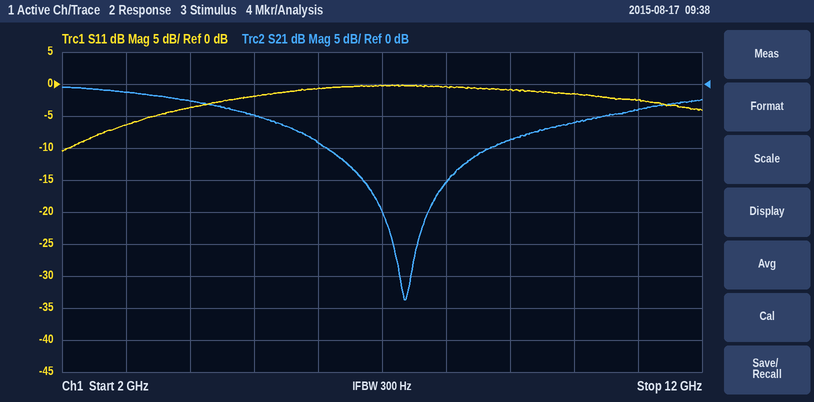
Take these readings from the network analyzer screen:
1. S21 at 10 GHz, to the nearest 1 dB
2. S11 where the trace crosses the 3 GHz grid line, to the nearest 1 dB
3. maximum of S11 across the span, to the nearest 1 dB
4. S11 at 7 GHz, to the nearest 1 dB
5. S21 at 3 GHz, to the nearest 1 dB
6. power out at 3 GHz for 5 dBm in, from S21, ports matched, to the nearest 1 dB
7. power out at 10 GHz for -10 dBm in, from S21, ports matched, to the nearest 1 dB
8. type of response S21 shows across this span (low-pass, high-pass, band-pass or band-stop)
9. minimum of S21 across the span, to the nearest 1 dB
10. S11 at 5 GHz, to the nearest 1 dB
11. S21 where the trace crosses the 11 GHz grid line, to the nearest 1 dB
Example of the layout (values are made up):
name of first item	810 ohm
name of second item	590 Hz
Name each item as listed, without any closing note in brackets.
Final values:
S21 at 10 GHz, to the nearest 1 dB	-6 dB
S11 where the trace crosses the 3 GHz grid line, to the nearest 1 dB	-6 dB
maximum of S11 across the span, to the nearest 1 dB	0 dB
S11 at 7 GHz, to the nearest 1 dB	0 dB
S21 at 3 GHz, to the nearest 1 dB	-1 dB
power out at 3 GHz for 5 dBm in, from S21, ports matched, to the nearest 1 dB	4 dBm
power out at 10 GHz for -10 dBm in, from S21, ports matched, to the nearest 1 dB	-16 dBm
type of response S21 shows across this span	band-stop
minimum of S21 across the span, to the nearest 1 dB	-34 dB
S11 at 5 GHz, to the nearest 1 dB	-2 dB
S21 where the trace crosses the 11 GHz grid line, to the nearest 1 dB	-4 dB
